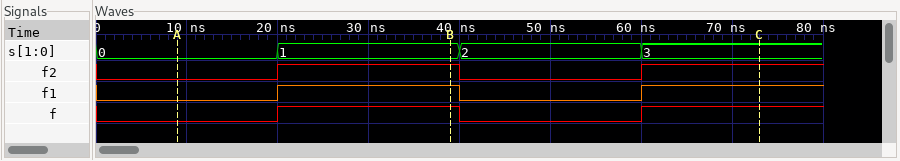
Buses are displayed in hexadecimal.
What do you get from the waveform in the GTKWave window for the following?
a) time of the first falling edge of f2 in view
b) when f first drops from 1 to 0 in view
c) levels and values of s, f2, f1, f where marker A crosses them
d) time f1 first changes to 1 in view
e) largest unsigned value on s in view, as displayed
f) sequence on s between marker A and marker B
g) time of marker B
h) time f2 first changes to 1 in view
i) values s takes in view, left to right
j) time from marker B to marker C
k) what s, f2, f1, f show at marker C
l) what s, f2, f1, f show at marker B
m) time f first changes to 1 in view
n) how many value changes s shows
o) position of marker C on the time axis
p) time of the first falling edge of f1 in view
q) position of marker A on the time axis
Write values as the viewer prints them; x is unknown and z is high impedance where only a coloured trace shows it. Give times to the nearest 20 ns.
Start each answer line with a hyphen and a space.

- 40 ns
- 40 ns
- s=0, f2=0, f1=0, f=0
- 20 ns
- 3
- 0, 1
- 40 ns
- 20 ns
- 0, 1, 2, 3
- 40 ns
- s=3, f2=1, f1=1, f=1
- s=1, f2=1, f1=1, f=1
- 20 ns
- 3
- 80 ns
- 40 ns
- 0 ns
